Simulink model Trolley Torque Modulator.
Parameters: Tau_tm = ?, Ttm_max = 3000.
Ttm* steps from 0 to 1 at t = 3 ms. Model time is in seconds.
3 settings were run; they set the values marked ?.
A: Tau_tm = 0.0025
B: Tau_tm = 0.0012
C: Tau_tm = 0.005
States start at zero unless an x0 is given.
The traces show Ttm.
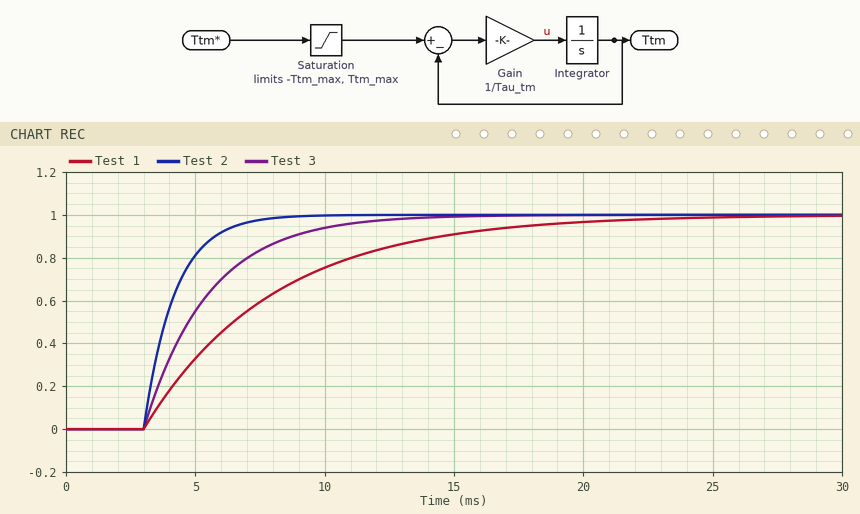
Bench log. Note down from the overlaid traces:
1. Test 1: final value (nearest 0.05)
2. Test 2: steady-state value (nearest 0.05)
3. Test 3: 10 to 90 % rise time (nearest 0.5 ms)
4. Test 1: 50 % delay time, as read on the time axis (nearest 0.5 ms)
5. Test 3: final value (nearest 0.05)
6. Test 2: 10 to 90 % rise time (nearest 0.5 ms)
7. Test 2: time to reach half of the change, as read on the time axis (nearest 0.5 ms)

1.00
1.00
5.5 ms
6.5 ms
1.00
2.5 ms
4.0 ms
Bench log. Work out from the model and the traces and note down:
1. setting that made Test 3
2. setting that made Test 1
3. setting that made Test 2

A
C
B
